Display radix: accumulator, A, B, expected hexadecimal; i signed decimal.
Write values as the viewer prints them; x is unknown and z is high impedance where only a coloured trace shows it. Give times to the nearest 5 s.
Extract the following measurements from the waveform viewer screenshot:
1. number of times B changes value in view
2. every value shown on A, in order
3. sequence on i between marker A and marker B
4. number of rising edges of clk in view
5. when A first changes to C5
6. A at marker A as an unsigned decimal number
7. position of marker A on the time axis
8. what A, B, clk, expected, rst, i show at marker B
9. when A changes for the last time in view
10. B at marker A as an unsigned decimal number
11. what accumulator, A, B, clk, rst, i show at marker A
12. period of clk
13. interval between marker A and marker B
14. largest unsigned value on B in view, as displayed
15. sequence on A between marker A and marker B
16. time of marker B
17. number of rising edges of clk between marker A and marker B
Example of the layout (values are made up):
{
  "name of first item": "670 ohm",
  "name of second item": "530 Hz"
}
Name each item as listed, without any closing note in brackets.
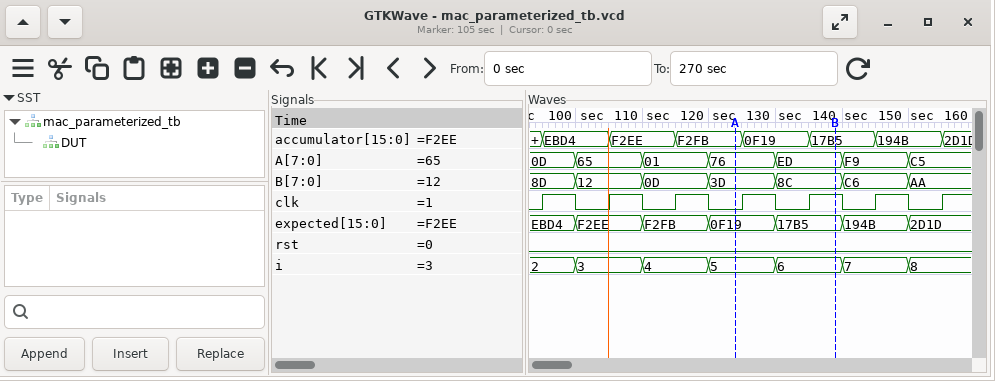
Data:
{
  "number of times B changes value in view": "6",
  "every value shown on A, in order": "0D, 65, 01, 76, ED, F9, C5",
  "sequence on i between marker A and marker B": "5, 6",
  "number of rising edges of clk in view": "7",
  "when A first changes to C5": "150 s",
  "A at marker A as an unsigned decimal number": "118",
  "position of marker A on the time axis": "125 s",
  "what A, B, clk, expected, rst, i show at marker B": "A=ED, B=8C, clk=1, expected=17B5, rst=0, i=6",
  "when A changes for the last time in view": "150 s",
  "B at marker A as an unsigned decimal number": "61",
  "what accumulator, A, B, clk, rst, i show at marker A": "accumulator=F2FB, A=76, B=3D, clk=0, rst=0, i=5",
  "period of clk": "10 s",
  "interval between marker A and marker B": "15 s",
  "largest unsigned value on B in view, as displayed": "C6",
  "sequence on A between marker A and marker B": "76, ED",
  "time of marker B": "140 s",
  "number of rising edges of clk between marker A and marker B": "2"
}
